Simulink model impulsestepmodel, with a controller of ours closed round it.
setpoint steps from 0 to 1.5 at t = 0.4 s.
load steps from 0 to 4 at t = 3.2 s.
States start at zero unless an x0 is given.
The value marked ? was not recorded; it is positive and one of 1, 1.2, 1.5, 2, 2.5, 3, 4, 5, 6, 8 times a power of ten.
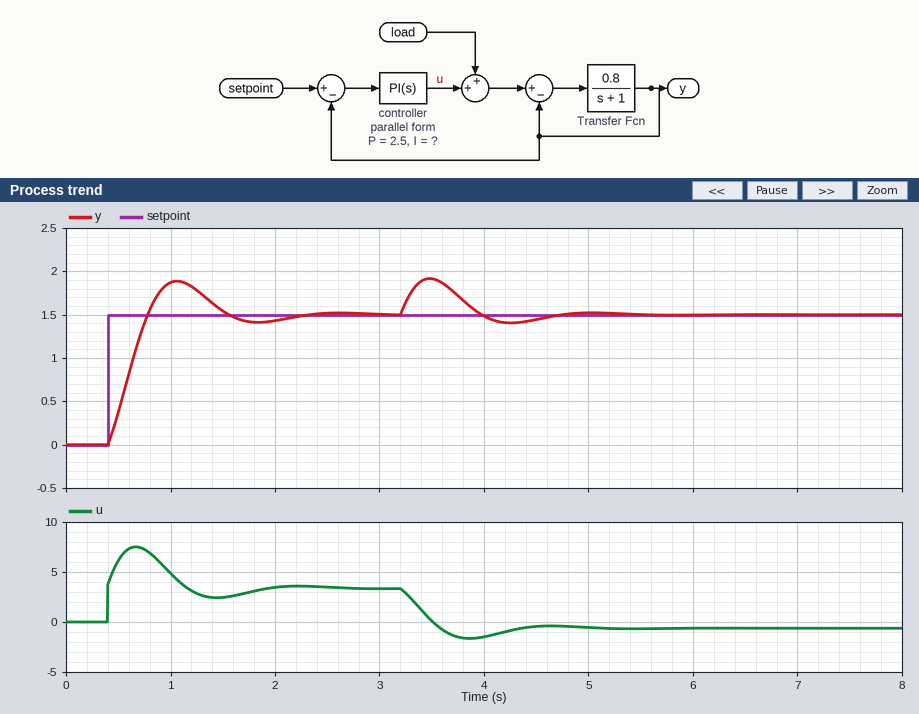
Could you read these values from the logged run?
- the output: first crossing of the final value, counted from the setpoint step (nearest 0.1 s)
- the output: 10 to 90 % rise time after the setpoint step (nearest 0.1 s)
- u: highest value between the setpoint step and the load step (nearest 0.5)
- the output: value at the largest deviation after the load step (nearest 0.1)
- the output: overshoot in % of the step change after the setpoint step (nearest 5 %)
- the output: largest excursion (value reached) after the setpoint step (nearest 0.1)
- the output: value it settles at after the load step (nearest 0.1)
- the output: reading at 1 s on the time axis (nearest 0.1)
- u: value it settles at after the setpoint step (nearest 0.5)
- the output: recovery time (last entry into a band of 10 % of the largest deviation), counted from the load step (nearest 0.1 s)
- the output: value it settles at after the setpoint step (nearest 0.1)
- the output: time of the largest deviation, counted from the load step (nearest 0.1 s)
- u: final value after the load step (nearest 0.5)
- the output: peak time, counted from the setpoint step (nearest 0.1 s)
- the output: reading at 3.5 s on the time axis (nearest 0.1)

0.4 s
0.3 s
7.5
1.9
25 %
1.9
1.5
1.9
3.5
1.4 s
1.5
0.3 s
-0.5
0.7 s
1.9
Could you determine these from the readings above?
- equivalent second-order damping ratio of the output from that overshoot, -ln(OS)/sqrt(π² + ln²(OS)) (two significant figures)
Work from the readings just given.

0.40
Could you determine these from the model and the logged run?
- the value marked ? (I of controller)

25
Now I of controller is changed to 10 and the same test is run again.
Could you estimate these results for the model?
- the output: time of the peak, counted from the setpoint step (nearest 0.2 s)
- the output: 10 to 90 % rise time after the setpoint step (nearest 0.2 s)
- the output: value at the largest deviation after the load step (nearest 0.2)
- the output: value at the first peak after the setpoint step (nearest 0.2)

1.2 s
0.6 s
2.0
1.6
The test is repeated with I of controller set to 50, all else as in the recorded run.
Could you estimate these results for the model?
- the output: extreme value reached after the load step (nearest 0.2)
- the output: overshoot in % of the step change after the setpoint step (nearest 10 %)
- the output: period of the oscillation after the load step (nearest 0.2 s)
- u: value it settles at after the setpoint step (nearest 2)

1.8
40 %
1.0 s
4
